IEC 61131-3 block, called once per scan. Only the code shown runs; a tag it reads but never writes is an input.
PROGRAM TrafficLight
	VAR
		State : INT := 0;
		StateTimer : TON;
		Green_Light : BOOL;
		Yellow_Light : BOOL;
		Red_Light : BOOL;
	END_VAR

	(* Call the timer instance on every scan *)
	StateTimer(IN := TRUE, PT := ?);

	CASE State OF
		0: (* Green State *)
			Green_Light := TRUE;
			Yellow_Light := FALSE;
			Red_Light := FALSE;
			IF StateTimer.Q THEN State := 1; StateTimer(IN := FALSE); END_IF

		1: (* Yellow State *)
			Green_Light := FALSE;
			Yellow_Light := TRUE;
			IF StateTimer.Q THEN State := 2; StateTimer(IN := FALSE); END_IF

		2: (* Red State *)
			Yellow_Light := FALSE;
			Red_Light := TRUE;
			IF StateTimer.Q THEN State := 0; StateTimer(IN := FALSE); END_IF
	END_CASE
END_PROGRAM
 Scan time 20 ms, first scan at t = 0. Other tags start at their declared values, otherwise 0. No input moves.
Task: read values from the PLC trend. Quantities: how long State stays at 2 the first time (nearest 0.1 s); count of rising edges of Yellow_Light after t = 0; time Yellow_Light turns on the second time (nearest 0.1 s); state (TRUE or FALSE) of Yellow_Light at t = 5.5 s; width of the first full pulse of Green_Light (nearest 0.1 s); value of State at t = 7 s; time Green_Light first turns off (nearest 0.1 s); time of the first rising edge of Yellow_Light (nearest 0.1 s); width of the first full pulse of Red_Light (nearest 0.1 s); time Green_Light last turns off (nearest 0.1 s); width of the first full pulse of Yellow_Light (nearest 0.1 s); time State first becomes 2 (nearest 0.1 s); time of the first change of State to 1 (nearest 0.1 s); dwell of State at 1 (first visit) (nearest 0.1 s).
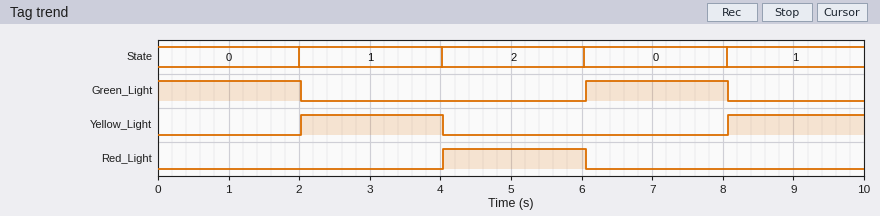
2.0 s
2
8.1 s
FALSE
2.0 s
0
2.0 s
2.0 s
2.0 s
8.1 s
2.0 s
4.0 s
2.0 s
2.0 s
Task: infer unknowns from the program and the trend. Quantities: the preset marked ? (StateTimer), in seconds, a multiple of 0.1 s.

2.0 s
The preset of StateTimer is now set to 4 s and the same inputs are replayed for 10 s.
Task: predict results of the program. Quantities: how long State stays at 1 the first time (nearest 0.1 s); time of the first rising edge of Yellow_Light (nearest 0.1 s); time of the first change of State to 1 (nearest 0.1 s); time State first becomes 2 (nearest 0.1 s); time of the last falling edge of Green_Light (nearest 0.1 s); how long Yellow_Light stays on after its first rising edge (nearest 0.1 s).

4.0 s
4.0 s
4.0 s
8.0 s
4.0 s
4.0 s
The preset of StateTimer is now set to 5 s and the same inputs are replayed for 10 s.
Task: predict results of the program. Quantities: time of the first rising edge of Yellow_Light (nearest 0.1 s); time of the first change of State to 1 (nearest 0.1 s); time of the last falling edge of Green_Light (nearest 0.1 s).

5.0 s
5.0 s
5.0 s
